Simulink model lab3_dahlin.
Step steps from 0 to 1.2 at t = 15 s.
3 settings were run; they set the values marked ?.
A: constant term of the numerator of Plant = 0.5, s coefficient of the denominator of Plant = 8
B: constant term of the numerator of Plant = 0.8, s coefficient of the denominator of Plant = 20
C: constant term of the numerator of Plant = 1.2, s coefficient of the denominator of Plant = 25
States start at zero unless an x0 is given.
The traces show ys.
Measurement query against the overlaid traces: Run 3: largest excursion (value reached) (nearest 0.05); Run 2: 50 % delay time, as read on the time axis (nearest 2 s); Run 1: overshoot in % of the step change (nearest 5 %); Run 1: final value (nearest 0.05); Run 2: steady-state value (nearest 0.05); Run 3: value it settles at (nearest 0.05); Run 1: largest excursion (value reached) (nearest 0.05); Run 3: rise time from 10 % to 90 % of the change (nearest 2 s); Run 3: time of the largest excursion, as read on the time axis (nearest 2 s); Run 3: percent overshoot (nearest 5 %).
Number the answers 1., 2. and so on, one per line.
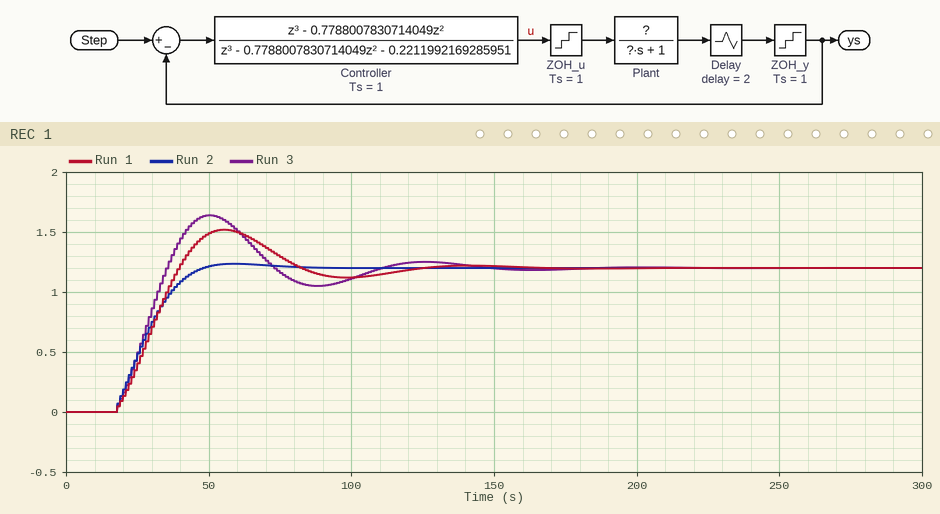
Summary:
1. 1.65
2. 28 s
3. 25 %
4. 1.20
5. 1.20
6. 1.20
7. 1.50
8. 14 s
9. 50 s
10. 35 %
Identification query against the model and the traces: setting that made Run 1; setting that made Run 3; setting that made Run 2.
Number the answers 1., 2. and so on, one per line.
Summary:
1. B
2. C
3. A
